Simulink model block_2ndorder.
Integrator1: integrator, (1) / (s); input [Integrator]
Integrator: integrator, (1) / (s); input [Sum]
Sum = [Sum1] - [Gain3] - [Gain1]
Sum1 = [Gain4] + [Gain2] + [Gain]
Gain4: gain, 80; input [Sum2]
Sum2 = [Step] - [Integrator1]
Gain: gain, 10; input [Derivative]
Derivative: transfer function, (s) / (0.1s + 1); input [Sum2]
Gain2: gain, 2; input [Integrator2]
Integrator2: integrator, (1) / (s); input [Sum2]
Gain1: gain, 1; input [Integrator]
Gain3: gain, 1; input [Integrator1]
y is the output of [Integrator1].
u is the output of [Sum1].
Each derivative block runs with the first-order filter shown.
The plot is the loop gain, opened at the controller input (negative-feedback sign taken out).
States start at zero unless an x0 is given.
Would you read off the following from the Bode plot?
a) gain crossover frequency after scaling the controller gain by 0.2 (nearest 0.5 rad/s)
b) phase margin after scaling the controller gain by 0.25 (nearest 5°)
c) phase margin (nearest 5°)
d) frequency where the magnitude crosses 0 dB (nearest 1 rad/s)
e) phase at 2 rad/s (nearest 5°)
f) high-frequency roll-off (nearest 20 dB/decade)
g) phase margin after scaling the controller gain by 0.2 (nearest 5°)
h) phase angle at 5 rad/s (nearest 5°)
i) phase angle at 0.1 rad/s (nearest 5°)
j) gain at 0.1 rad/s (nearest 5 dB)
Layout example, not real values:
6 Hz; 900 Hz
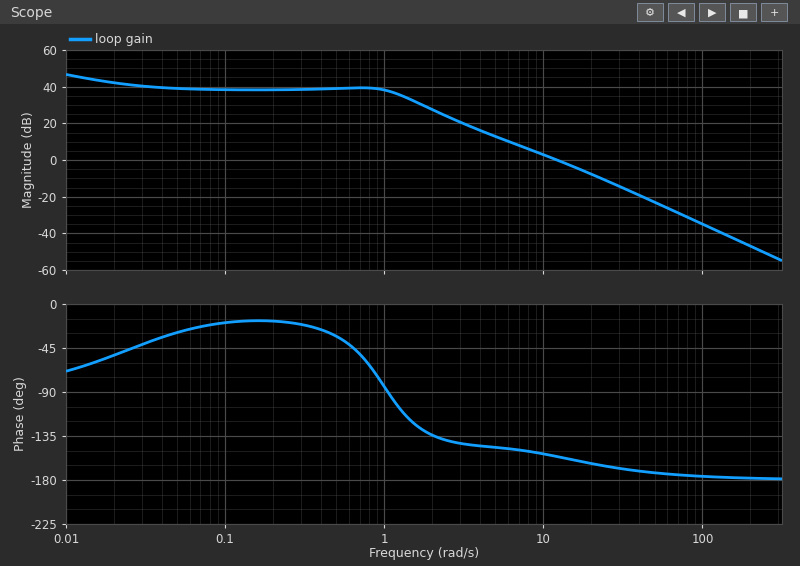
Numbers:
4.5 rad/s; 35°; 25°; 12 rad/s; -135°; -40 dB/decade; 35°; -145°; -20°; 40 dB
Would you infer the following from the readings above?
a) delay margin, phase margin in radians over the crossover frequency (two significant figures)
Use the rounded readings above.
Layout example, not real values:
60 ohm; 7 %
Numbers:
0.036 s
